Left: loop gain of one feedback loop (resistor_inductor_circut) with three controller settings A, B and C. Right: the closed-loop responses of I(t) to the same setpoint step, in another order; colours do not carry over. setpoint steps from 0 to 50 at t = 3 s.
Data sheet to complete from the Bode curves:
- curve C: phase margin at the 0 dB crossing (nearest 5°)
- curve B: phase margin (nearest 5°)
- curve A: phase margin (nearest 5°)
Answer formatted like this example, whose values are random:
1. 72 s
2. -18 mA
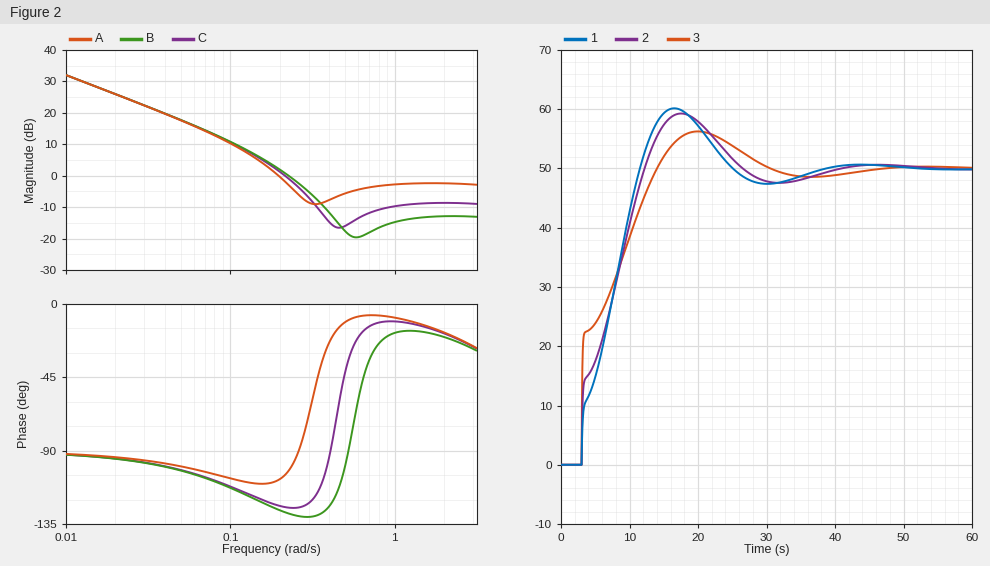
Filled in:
1. 55°
2. 50°
3. 70°
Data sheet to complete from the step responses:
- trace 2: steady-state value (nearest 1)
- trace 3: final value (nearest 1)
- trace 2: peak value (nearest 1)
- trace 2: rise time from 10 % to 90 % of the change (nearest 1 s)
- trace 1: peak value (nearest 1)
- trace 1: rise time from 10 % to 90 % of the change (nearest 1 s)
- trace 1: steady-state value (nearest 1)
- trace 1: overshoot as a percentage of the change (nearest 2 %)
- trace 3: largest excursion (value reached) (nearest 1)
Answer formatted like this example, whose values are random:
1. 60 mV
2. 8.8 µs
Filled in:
1. 50
2. 50
3. 59
4. 8 s
5. 60
6. 7 s
7. 50
8. 20 %
9. 56
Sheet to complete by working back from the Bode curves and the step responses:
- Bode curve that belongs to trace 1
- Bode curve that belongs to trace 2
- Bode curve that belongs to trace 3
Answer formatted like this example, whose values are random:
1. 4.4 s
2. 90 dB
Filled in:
1. B
2. C
3. A
